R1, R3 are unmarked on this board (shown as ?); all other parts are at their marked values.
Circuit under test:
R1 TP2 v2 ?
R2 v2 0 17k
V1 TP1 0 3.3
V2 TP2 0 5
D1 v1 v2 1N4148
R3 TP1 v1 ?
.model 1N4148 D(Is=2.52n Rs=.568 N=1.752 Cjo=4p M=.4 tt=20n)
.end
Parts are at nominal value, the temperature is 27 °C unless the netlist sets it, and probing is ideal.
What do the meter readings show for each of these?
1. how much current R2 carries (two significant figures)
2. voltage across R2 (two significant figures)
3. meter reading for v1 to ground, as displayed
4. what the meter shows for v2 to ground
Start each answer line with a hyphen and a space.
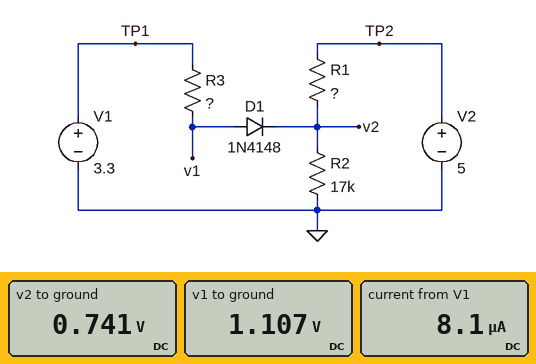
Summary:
- 44 µA
- 740 mV
- 1.107 V
- 0.741 V
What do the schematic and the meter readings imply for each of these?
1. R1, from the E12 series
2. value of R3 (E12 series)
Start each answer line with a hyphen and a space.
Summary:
- 120 kΩ
- 270 kΩ
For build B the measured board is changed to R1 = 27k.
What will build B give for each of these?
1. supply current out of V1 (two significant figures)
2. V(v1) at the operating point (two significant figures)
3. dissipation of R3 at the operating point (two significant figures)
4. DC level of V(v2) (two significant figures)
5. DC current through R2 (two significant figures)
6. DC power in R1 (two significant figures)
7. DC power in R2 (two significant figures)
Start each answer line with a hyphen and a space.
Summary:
- 3.7 µA
- 2.3 V
- 3.7 µW
- 2.0 V
- 120 µA
- 340 µW
- 230 µW
